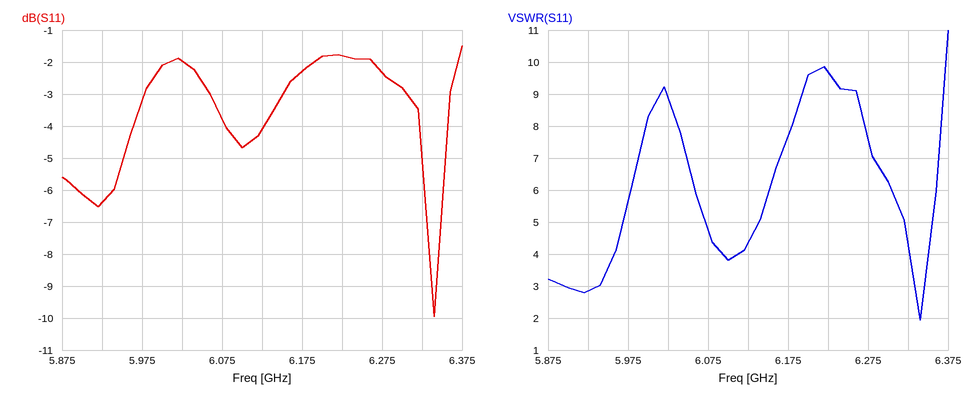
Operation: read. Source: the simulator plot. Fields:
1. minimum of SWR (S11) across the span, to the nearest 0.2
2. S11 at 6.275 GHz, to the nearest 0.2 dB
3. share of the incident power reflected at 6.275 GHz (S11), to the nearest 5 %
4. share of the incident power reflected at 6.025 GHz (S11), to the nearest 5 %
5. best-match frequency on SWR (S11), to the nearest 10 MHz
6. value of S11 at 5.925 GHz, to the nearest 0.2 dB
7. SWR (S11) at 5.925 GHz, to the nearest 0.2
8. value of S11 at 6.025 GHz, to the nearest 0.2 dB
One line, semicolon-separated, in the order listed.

2.0; -2.4 dB; 60 %; 65 %; 6.34 GHz; -6.4 dB; 2.8; -2.0 dB
